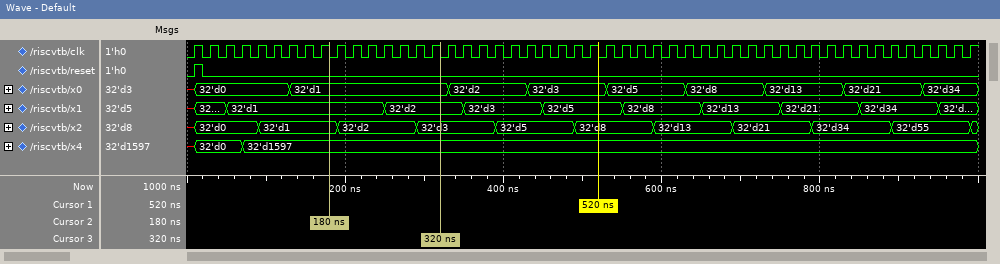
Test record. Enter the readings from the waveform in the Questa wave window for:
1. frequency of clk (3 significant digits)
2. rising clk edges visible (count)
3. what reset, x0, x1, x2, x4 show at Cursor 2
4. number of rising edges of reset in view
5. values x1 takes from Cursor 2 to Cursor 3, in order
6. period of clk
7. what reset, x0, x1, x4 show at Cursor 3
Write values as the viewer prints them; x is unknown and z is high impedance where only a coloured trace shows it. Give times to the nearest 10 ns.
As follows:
50.0 MHz
50
reset=0, x0=32'd1, x1=32'd1, x2=32'd1, x4=32'd1597
1
32'd1, 32'd2
20 ns
reset=0, x0=32'd1, x1=32'd2, x4=32'd1597
